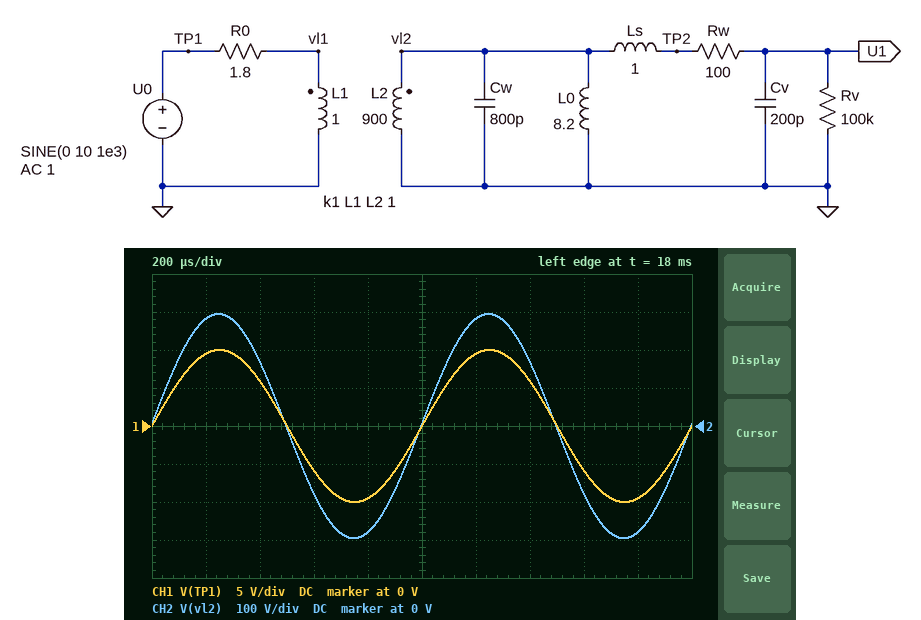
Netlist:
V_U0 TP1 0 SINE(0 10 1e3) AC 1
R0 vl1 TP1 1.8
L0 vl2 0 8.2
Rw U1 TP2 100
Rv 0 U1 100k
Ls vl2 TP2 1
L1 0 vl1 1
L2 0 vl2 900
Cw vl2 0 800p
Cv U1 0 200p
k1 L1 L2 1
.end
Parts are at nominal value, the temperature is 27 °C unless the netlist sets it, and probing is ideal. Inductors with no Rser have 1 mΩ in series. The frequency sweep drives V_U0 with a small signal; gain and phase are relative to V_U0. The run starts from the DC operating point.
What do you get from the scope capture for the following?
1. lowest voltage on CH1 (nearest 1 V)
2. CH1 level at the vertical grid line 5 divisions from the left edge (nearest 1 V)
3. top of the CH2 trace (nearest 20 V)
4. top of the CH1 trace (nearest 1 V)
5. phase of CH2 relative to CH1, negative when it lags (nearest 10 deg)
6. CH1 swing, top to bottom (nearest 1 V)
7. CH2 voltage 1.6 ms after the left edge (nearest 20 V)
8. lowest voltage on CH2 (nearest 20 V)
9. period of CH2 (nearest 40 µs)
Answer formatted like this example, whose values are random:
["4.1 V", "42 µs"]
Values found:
["-10 V", "0 V", "300 V", "10 V", "0 deg", "20 V", "-180 V", "-300 V", "1.00 ms"]
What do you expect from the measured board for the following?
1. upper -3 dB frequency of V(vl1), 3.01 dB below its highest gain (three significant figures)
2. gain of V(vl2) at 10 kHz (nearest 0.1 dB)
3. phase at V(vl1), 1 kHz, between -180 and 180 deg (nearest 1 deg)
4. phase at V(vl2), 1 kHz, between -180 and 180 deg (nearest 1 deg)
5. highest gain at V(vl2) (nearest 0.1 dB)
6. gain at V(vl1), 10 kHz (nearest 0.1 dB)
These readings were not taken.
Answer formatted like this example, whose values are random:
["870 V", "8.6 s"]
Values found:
["126 kHz", "29.2 dB", "1 deg", "1 deg", "29.4 dB", "-0.3 dB"]
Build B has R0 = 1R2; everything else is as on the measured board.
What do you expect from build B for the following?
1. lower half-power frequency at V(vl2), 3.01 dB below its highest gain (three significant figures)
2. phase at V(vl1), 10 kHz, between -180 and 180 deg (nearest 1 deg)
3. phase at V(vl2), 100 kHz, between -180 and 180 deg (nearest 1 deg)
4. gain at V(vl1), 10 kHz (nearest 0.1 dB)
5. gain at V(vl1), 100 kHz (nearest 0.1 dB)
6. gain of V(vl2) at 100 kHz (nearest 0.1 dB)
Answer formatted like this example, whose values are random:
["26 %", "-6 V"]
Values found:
["21.1 Hz", "-2 deg", "-28 deg", "-0.2 dB", "-1.1 dB", "28.4 dB"]
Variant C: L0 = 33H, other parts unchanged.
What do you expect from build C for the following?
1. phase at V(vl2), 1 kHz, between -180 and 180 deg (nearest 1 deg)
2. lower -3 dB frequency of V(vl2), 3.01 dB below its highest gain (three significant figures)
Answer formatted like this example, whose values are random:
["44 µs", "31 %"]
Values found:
["0 deg", "8.04 Hz"]
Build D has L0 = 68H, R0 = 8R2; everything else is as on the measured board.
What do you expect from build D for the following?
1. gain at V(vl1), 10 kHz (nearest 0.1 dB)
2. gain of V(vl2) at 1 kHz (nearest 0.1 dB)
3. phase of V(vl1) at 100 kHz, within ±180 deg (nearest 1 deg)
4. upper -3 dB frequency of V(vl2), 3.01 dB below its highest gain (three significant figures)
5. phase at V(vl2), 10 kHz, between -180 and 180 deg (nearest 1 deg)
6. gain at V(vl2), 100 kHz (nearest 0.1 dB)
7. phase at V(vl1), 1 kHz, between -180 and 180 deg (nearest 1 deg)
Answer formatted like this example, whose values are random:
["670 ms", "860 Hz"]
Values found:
["-1.6 dB", "28.9 dB", "-75 deg", "31.9 kHz", "-15 deg", "17.9 dB", "-1 deg"]
